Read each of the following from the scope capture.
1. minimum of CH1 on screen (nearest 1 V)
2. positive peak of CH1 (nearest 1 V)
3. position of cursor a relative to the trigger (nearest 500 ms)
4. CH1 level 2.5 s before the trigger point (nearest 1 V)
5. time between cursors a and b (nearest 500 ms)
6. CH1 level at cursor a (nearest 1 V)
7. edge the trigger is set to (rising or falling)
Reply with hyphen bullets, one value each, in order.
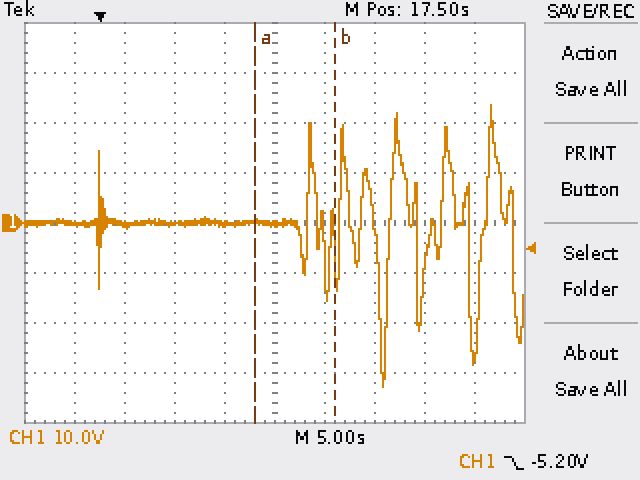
- -33 V
- 24 V
- +15.5 s
- 0 V
- 8.0 s
- 0 V
- falling
